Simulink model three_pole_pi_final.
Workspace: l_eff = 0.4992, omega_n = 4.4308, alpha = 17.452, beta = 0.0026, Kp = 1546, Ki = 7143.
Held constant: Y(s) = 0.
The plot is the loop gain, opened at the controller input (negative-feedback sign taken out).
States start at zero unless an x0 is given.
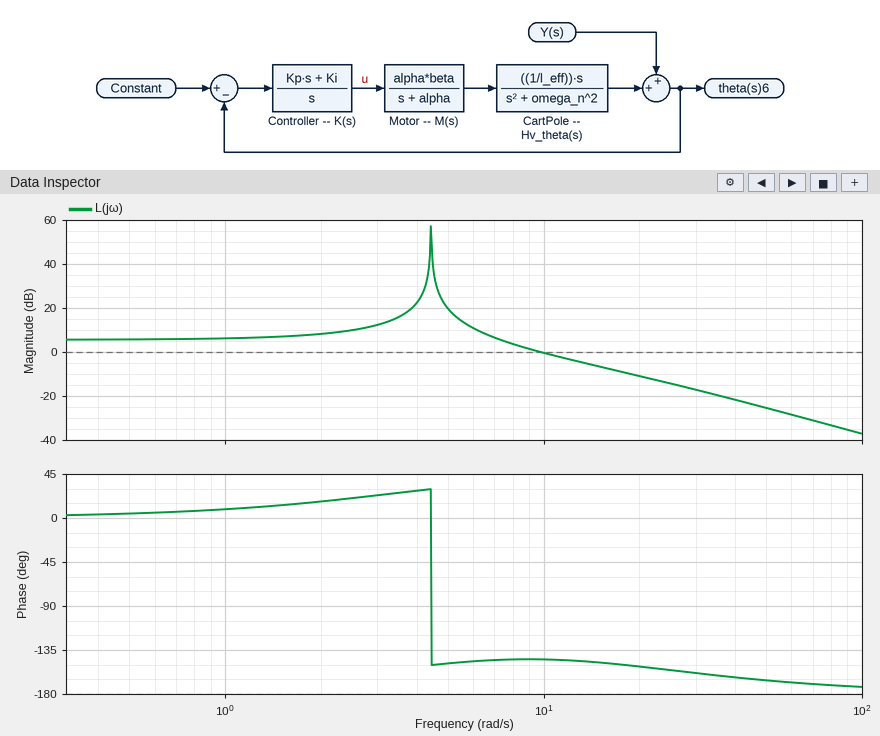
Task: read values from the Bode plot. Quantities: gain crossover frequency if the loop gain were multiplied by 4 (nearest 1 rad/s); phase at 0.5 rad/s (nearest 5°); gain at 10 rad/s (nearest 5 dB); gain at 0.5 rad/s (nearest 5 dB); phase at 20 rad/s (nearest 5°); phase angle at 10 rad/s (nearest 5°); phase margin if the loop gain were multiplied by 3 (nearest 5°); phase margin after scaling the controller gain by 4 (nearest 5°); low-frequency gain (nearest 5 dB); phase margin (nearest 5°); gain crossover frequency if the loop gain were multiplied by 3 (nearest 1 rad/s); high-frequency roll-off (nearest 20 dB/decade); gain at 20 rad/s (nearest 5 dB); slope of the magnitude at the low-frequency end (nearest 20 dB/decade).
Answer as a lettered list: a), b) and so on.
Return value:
a) 22 rad/s
b) 5°
c) 0 dB
d) 5 dB
e) -150°
f) -145°
g) 30°
h) 25°
i) 5 dB
j) 35°
k) 18 rad/s
l) -40 dB/decade
m) -10 dB
n) 0 dB/decade
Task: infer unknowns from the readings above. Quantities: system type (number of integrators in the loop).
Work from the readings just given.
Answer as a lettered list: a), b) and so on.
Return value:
a) 0
